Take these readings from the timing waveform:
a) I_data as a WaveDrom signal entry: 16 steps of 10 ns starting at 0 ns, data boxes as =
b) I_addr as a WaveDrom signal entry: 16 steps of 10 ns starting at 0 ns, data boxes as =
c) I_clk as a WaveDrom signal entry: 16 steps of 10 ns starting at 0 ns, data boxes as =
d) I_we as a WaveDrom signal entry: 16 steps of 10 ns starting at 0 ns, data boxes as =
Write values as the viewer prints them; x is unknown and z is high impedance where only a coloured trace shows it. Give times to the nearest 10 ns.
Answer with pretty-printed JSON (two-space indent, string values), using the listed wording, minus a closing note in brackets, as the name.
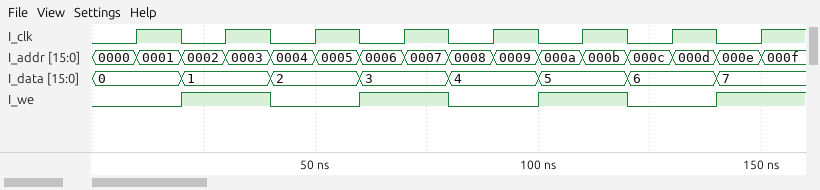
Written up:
{
  "I_data as a WaveDrom signal entry: 16 steps of 10 ns starting at 0 ns, data boxes as =": "{name: 'I_data', wave: '=.=.=.=.=.=.=.=.', data: '0 1 2 3 4 5 6 7'}",
  "I_addr as a WaveDrom signal entry: 16 steps of 10 ns starting at 0 ns, data boxes as =": "{name: 'I_addr', wave: '================', data: '0000 0001 0002 0003 0004 0005 0006 0007 0008 0009 000a 000b 000c 000d 000e 000f'}",
  "I_clk as a WaveDrom signal entry: 16 steps of 10 ns starting at 0 ns, data boxes as =": "{name: 'I_clk', wave: '0101010101010101'}",
  "I_we as a WaveDrom signal entry: 16 steps of 10 ns starting at 0 ns, data boxes as =": "{name: 'I_we', wave: '0.1.0.1.0.1.0.1.'}"
}
